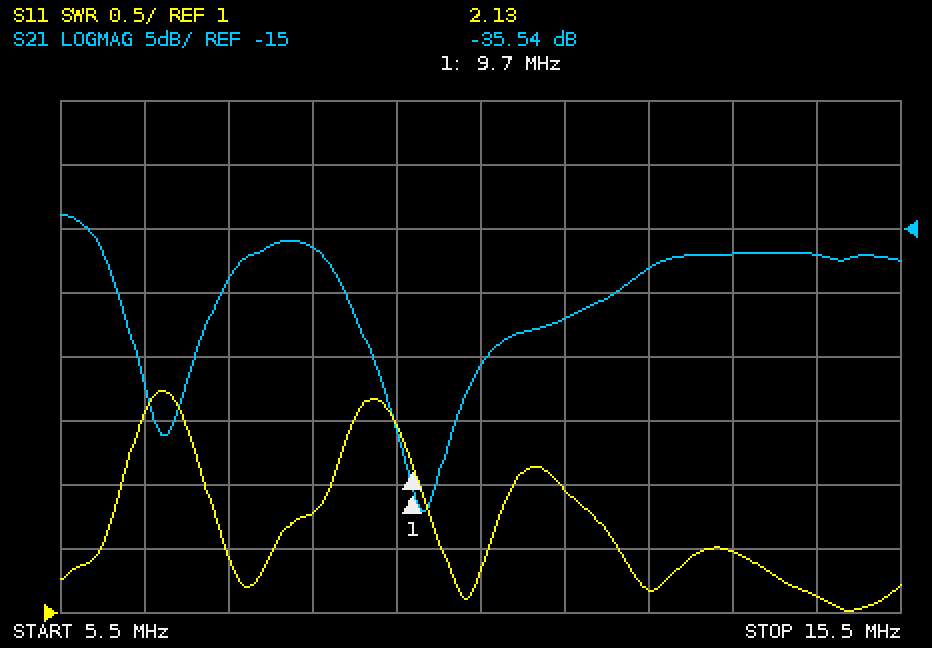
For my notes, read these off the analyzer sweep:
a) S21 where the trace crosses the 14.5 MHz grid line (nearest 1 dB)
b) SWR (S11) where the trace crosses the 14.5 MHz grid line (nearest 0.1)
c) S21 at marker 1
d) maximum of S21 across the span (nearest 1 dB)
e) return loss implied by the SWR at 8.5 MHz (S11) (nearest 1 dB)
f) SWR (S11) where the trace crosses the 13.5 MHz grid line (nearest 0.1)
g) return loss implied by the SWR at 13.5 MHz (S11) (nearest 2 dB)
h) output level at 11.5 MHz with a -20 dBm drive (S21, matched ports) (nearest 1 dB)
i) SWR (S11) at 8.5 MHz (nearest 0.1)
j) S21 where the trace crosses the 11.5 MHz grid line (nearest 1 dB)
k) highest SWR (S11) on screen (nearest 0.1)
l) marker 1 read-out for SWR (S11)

-17 dB
1.1
-35.54 dB
-14 dB
11 dB
1.5
14 dB
-42 dBm
1.8
-22 dB
2.7
2.13
